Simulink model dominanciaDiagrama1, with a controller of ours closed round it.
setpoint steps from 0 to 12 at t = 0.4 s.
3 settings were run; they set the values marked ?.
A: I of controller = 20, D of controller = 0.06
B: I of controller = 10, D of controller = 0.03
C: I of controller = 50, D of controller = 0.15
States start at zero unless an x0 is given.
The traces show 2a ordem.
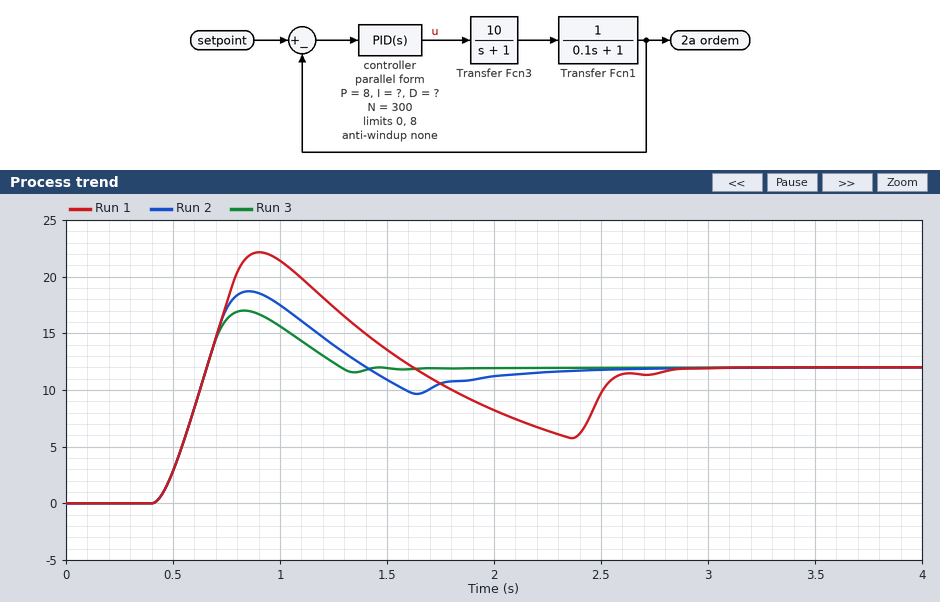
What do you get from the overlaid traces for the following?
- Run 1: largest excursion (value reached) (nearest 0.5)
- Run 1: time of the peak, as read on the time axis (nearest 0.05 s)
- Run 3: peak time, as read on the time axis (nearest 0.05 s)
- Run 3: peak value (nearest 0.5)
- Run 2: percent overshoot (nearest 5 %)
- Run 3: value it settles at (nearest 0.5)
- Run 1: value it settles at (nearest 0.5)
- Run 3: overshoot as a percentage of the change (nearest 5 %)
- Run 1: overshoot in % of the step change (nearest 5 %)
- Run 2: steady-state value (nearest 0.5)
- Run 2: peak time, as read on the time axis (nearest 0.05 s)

22.0
0.90 s
0.85 s
17.0
55 %
12.0
12.0
40 %
85 %
12.0
0.85 s
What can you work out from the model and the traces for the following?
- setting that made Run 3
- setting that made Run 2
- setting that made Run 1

B
A
C
